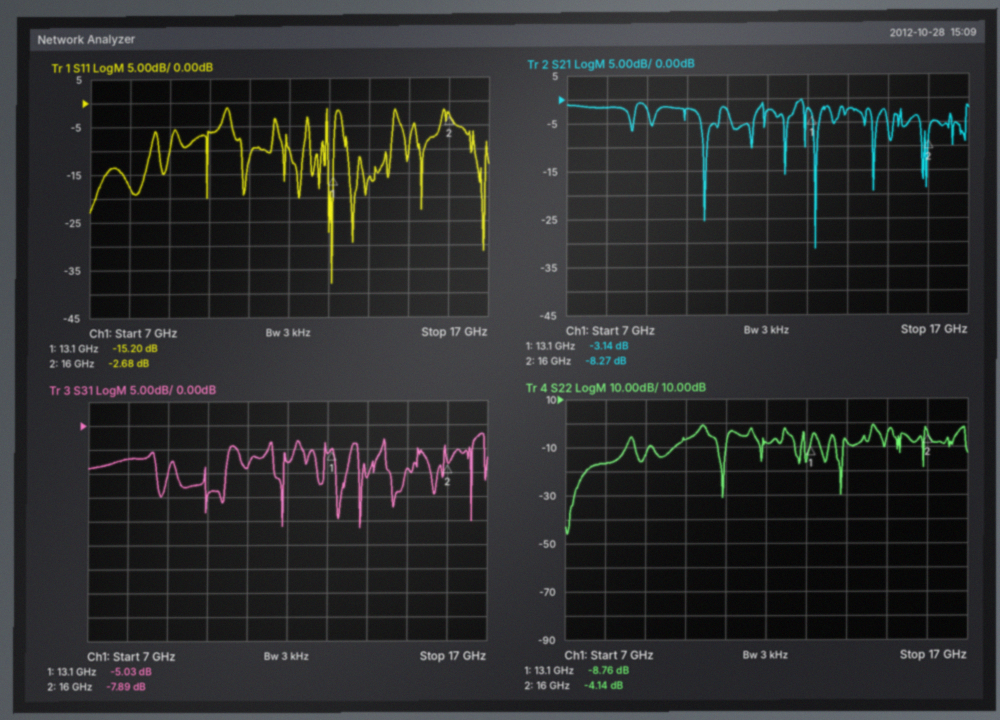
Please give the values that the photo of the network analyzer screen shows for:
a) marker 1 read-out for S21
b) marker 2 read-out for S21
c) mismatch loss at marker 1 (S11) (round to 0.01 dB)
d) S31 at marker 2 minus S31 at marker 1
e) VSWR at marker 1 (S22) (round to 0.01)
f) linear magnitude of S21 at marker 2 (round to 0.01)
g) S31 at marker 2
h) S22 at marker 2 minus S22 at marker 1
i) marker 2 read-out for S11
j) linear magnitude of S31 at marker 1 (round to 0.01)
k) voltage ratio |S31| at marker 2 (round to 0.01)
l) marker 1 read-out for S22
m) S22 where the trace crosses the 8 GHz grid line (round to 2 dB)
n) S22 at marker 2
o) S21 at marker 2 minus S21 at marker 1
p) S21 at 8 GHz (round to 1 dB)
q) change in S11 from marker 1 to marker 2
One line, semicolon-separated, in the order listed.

-3.14 dB; -8.27 dB; 0.13 dB; -2.86 dB; 2.15; 0.39; -7.89 dB; 4.62 dB; -2.68 dB; 0.56; 0.40; -8.76 dB; -16 dB; -4.14 dB; -5.13 dB; -2 dB; 12.52 dB
